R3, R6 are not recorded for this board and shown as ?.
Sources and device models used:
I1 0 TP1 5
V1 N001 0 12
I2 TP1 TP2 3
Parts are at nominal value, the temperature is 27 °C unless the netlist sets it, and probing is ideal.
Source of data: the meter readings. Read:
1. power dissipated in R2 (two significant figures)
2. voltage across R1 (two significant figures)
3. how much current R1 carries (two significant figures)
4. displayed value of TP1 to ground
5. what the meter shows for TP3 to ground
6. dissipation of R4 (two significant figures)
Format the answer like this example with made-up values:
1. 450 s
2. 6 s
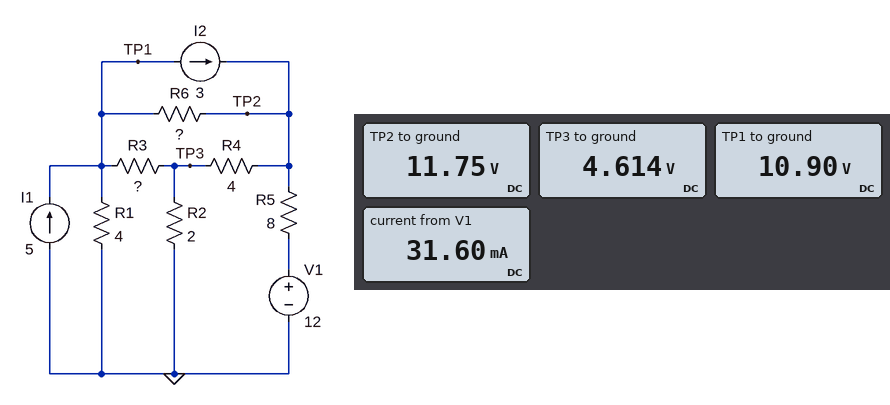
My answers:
1. 11 W
2. 11 V
3. 2.7 A
4. 10.90 V
5. 4.614 V
6. 13 W
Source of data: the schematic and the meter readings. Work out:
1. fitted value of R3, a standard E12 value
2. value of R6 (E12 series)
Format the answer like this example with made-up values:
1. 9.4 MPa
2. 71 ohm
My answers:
1. 12 Ω
2. 0.68 Ω
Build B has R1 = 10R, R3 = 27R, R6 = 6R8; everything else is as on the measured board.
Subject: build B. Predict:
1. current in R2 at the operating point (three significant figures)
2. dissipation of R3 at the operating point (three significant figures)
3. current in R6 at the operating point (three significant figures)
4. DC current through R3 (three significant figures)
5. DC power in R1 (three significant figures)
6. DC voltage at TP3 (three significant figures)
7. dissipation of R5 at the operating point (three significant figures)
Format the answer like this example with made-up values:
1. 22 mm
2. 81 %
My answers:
1. 2.91 A
2. 3.87 W
3. 17.3 mA
4. 379 mA
5. 25.7 W
6. 5.81 V
7. 1.92 W
